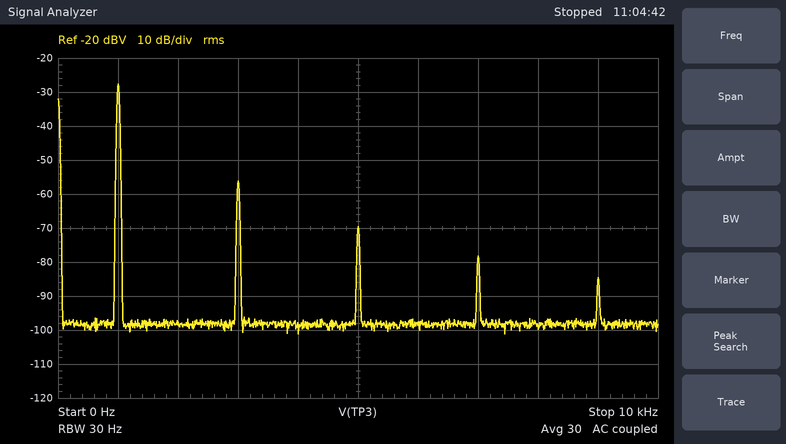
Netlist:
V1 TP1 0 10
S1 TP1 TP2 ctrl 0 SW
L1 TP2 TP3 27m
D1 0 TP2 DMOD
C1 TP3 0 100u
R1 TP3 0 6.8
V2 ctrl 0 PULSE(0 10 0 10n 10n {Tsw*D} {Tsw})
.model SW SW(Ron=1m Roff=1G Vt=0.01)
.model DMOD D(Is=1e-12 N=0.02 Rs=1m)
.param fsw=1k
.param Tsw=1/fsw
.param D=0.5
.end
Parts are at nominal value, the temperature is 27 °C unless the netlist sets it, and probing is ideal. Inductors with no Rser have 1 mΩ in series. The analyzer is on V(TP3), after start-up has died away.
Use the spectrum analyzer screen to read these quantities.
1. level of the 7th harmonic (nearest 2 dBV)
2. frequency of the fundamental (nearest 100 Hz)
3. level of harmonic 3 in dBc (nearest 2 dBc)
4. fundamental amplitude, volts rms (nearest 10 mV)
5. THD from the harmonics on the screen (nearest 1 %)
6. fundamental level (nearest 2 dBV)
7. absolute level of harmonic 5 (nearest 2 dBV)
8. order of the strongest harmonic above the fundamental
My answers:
-78 dBV
1.0 kHz
-28 dBc
40 mV
4 %
-28 dBV
-70 dBV
3
